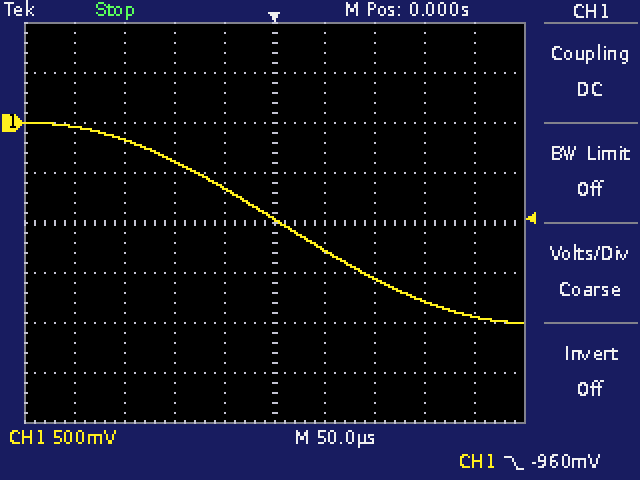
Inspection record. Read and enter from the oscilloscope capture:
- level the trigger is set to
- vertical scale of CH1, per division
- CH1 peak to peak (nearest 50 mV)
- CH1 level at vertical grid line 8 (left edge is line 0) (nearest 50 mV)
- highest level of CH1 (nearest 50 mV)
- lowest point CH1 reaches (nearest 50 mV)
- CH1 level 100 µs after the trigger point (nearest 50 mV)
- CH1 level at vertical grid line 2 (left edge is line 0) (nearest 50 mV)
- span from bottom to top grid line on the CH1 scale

-960 mV
500 mV
2.00 V
-1.80 V
0 mV
-2.00 V
-1.55 V
-150 mV
4 V
